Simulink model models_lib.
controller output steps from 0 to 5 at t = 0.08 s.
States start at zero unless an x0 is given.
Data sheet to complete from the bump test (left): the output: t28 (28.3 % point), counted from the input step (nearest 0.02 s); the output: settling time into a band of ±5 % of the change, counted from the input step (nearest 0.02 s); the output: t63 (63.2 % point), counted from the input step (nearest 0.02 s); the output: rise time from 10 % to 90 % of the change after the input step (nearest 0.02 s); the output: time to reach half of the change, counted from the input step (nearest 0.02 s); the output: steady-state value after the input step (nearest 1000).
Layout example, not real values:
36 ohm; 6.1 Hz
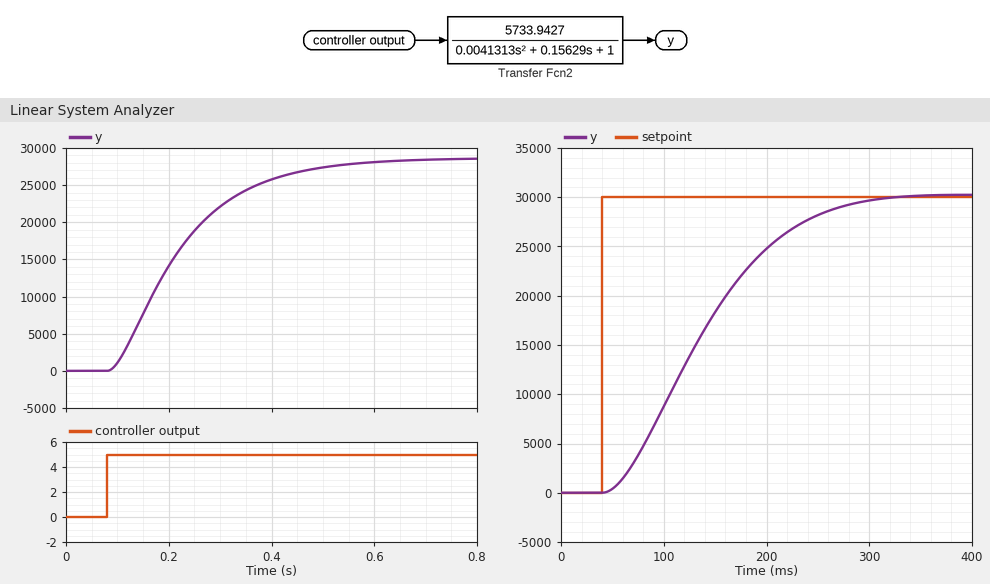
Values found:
0.08 s; 0.40 s; 0.16 s; 0.28 s; 0.12 s; 29000
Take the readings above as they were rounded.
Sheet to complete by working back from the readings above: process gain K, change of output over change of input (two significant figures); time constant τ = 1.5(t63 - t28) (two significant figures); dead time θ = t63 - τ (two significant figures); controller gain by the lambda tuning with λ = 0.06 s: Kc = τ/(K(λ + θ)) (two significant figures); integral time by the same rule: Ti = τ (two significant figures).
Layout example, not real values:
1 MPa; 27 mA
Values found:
5800; 0.12 s; 0.040 s; 0.00021; 0.12 s
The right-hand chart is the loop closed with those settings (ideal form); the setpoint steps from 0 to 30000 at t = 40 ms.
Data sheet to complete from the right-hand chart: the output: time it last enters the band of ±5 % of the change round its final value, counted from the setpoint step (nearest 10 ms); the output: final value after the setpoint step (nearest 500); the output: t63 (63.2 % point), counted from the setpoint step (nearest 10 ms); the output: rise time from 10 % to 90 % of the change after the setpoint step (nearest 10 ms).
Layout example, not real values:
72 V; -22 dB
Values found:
220 ms; 30000; 110 ms; 160 ms
